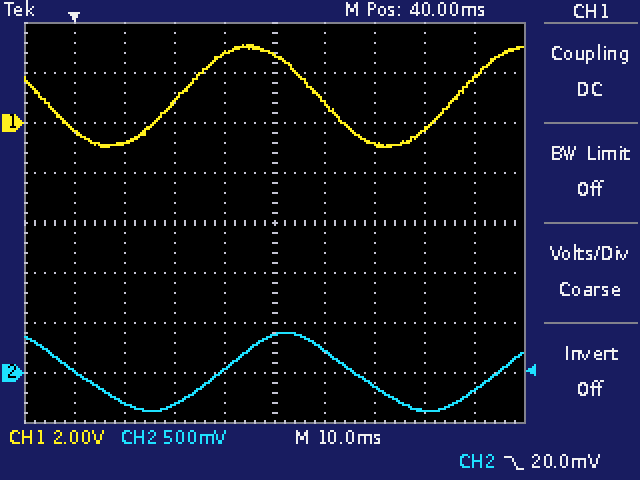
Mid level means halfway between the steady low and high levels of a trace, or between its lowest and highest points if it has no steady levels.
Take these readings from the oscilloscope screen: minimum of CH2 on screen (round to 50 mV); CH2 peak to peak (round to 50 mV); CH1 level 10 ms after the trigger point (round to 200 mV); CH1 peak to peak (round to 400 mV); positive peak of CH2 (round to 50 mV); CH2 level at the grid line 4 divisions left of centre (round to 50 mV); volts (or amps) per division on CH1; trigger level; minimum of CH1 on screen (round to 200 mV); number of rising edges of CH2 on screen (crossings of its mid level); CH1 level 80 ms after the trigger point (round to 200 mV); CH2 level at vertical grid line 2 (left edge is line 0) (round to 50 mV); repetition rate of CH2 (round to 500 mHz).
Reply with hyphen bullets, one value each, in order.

- -400 mV
- 800 mV
- -800 mV
- 4.0 V
- 400 mV
- 0 mV
- 2 V
- 20.0 mV
- -1.0 V
- 2
- 1.8 V
- -300 mV
- 18.0 Hz
